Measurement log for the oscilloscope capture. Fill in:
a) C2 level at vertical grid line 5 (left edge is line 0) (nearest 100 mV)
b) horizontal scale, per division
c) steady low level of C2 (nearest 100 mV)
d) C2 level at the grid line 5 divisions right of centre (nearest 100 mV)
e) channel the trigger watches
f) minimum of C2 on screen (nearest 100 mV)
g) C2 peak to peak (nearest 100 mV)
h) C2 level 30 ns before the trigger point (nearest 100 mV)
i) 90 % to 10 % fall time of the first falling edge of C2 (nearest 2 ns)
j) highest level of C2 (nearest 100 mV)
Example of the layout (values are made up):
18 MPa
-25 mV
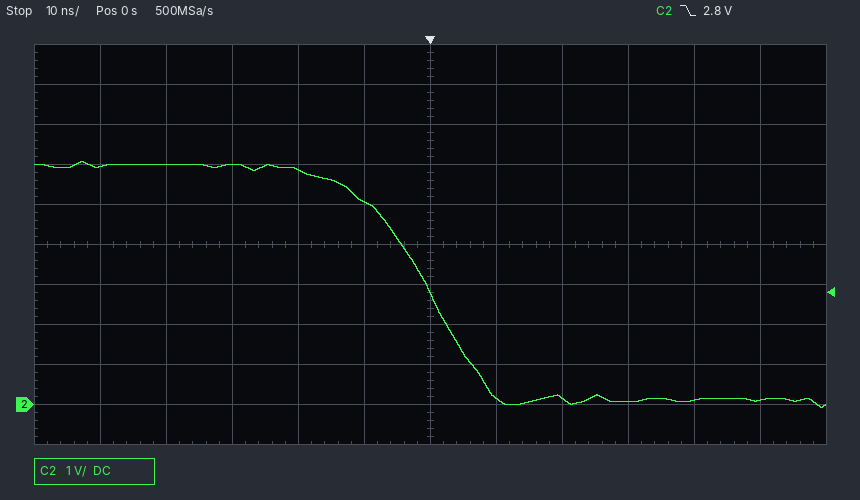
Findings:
5.1 V
10 ns
100 mV
100 mV
C2
-100 mV
6.2 V
6.0 V
20 ns
6.1 V
